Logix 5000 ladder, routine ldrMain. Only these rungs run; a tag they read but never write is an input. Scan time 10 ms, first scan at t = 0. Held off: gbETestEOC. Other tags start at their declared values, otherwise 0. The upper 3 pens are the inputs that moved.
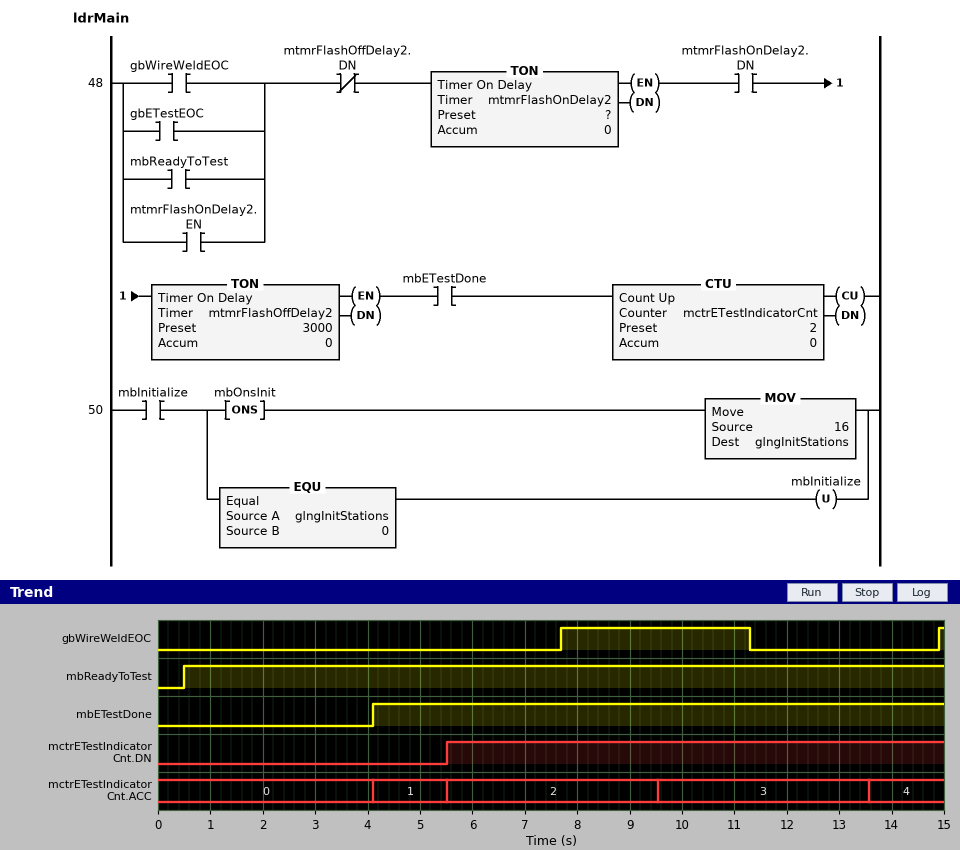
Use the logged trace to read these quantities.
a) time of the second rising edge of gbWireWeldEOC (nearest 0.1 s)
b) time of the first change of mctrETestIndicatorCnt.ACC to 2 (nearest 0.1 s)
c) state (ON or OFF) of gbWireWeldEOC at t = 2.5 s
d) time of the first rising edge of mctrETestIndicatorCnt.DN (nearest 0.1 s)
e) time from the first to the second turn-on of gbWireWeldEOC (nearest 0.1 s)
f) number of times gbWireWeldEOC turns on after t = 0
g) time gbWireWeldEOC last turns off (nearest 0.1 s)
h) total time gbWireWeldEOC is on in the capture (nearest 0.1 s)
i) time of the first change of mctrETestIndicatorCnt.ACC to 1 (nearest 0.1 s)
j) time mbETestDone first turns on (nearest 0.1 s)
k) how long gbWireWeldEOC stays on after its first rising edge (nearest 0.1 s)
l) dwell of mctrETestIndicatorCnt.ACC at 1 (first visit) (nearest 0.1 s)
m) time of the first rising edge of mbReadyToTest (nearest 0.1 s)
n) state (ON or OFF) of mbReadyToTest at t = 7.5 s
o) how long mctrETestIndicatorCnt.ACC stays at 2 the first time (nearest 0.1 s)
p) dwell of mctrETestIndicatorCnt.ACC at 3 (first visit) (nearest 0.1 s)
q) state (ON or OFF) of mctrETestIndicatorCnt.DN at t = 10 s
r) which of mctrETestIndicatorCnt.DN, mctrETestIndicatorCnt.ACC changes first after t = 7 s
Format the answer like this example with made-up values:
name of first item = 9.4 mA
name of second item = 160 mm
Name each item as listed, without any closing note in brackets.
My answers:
time of the second rising edge of gbWireWeldEOC = 14.9 s
time of the first change of mctrETestIndicatorCnt.ACC to 2 = 5.5 s
state (ON or OFF) of gbWireWeldEOC at t = 2.5 s = OFF
time of the first rising edge of mctrETestIndicatorCnt.DN = 5.5 s
time from the first to the second turn-on of gbWireWeldEOC = 7.2 s
number of times gbWireWeldEOC turns on after t = 0 = 2
time gbWireWeldEOC last turns off = 11.3 s
total time gbWireWeldEOC is on in the capture = 3.7 s
time of the first change of mctrETestIndicatorCnt.ACC to 1 = 4.1 s
time mbETestDone first turns on = 4.1 s
how long gbWireWeldEOC stays on after its first rising edge = 3.6 s
dwell of mctrETestIndicatorCnt.ACC at 1 (first visit) = 1.4 s
time of the first rising edge of mbReadyToTest = 0.5 s
state (ON or OFF) of mbReadyToTest at t = 7.5 s = ON
how long mctrETestIndicatorCnt.ACC stays at 2 the first time = 4.0 s
dwell of mctrETestIndicatorCnt.ACC at 3 (first visit) = 4.0 s
state (ON or OFF) of mctrETestIndicatorCnt.DN at t = 10 s = ON
which of mctrETestIndicatorCnt.DN, mctrETestIndicatorCnt.ACC changes first after t = 7 s = mctrETestIndicatorCnt.ACC
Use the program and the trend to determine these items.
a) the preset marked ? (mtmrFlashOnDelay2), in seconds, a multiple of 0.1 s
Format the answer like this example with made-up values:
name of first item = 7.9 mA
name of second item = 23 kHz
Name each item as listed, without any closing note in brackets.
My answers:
the preset marked ? (mtmrFlashOnDelay2), in seconds, a multiple of 0.1 s = 1.0 s
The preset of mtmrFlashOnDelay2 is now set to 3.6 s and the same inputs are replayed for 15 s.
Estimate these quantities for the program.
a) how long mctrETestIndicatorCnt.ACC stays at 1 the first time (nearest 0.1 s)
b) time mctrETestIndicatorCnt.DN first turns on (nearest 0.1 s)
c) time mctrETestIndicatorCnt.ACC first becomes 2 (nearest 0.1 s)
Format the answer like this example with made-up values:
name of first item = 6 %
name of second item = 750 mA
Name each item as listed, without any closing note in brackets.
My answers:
how long mctrETestIndicatorCnt.ACC stays at 1 the first time = 6.6 s
time mctrETestIndicatorCnt.DN first turns on = 10.7 s
time mctrETestIndicatorCnt.ACC first becomes 2 = 10.7 s
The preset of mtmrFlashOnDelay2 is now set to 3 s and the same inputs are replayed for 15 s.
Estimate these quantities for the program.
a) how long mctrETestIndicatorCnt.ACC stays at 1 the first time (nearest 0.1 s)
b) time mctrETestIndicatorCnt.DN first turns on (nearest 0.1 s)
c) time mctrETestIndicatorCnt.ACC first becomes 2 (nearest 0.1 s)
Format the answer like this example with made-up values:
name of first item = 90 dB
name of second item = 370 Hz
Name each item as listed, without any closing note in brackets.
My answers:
how long mctrETestIndicatorCnt.ACC stays at 1 the first time = 5.4 s
time mctrETestIndicatorCnt.DN first turns on = 9.5 s
time mctrETestIndicatorCnt.ACC first becomes 2 = 9.5 s
